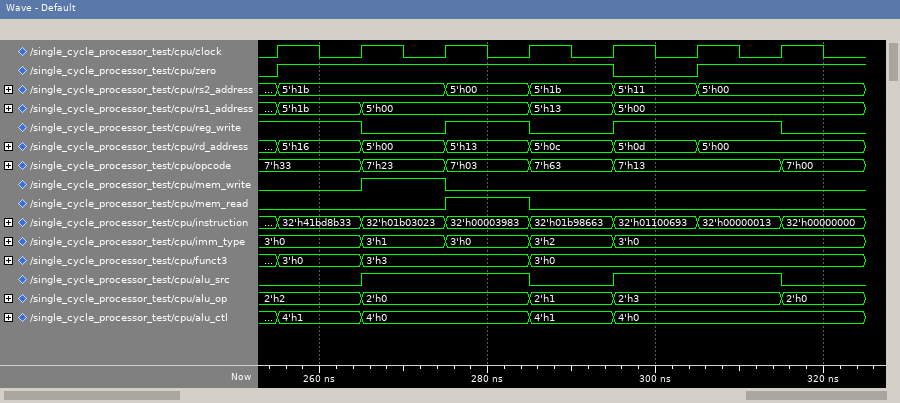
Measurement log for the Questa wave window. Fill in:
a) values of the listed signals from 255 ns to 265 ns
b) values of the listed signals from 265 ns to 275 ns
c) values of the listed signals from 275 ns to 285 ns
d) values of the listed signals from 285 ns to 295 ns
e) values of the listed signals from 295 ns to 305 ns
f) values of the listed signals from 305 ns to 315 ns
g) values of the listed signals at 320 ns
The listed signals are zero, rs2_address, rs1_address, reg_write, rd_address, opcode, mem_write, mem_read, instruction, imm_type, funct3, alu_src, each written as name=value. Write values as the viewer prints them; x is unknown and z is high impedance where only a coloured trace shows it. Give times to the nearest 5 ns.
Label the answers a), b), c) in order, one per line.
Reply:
a) zero=1, rs2_address=5'h1b, rs1_address=5'h1b, reg_write=1, rd_address=5'h16, opcode=7'h33, mem_write=0, mem_read=0, instruction=32'h41bd8b33, imm_type=3'h0, funct3=3'h0, alu_src=0
b) zero=1, rs2_address=5'h1b, rs1_address=5'h00, reg_write=0, rd_address=5'h00, opcode=7'h23, mem_write=1, mem_read=0, instruction=32'h01b03023, imm_type=3'h1, funct3=3'h3, alu_src=1
c) zero=1, rs2_address=5'h00, rs1_address=5'h00, reg_write=1, rd_address=5'h13, opcode=7'h03, mem_write=0, mem_read=1, instruction=32'h00003983, imm_type=3'h0, funct3=3'h3, alu_src=1
d) zero=1, rs2_address=5'h1b, rs1_address=5'h13, reg_write=0, rd_address=5'h0c, opcode=7'h63, mem_write=0, mem_read=0, instruction=32'h01b98663, imm_type=3'h2, funct3=3'h0, alu_src=0
e) zero=0, rs2_address=5'h11, rs1_address=5'h00, reg_write=1, rd_address=5'h0d, opcode=7'h13, mem_write=0, mem_read=0, instruction=32'h01100693, imm_type=3'h0, funct3=3'h0, alu_src=1
f) zero=1, rs2_address=5'h00, rs1_address=5'h00, reg_write=1, rd_address=5'h00, opcode=7'h13, mem_write=0, mem_read=0, instruction=32'h00000013, imm_type=3'h0, funct3=3'h0, alu_src=1
g) zero=1, rs2_address=5'h00, rs1_address=5'h00, reg_write=0, rd_address=5'h00, opcode=7'h00, mem_write=0, mem_read=0, instruction=32'h00000000, imm_type=3'h0, funct3=3'h0, alu_src=0
